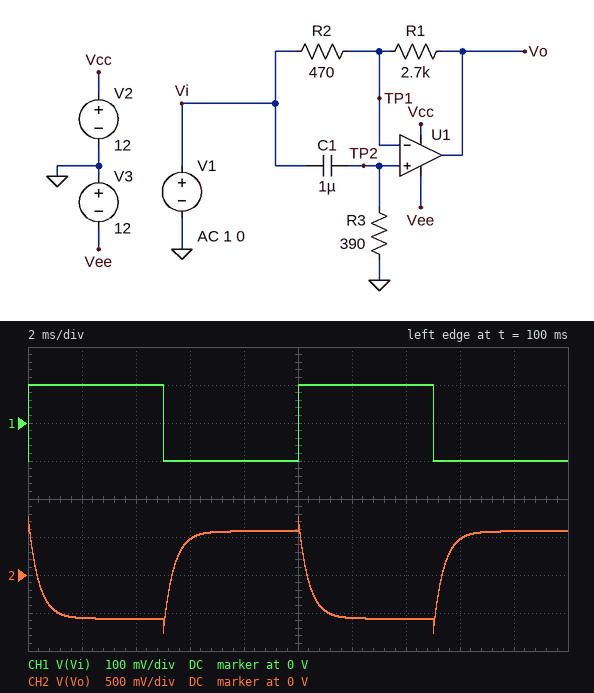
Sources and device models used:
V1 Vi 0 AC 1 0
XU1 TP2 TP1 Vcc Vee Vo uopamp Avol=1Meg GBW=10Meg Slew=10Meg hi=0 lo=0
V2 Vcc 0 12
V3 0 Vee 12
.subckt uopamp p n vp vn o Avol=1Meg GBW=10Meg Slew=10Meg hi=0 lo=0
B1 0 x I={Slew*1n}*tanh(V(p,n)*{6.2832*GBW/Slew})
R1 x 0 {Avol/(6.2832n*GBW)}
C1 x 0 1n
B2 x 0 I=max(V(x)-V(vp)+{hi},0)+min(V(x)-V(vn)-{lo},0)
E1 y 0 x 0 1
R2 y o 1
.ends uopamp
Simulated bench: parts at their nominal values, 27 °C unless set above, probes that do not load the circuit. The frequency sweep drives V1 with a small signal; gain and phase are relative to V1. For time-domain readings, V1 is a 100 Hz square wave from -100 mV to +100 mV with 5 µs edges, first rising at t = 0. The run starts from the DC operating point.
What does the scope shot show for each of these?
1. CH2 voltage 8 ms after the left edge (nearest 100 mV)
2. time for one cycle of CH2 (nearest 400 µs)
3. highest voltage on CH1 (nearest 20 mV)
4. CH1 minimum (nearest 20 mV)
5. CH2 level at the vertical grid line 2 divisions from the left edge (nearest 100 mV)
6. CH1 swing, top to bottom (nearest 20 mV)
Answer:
600 mV
10.0 ms
100 mV
-100 mV
-600 mV
200 mV
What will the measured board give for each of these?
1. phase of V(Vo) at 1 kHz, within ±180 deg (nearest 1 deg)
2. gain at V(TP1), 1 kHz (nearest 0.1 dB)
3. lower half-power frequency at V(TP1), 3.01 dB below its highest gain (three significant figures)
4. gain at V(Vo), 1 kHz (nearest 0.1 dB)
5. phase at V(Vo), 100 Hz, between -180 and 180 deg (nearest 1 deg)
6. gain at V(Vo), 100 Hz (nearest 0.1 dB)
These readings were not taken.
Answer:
89 deg
-0.7 dB
408 Hz
7.5 dB
164 deg
14.9 dB
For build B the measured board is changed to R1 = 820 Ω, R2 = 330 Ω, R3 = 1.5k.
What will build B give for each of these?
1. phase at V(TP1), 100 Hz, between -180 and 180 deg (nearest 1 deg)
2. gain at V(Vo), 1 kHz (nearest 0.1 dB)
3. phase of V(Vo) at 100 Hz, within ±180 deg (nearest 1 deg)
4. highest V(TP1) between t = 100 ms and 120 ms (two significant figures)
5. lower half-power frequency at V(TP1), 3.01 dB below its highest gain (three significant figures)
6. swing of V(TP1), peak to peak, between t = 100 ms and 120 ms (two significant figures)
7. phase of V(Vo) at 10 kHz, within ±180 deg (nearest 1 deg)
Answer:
47 deg
0.2 dB
116 deg
190 mV
106 Hz
390 mV
2 deg
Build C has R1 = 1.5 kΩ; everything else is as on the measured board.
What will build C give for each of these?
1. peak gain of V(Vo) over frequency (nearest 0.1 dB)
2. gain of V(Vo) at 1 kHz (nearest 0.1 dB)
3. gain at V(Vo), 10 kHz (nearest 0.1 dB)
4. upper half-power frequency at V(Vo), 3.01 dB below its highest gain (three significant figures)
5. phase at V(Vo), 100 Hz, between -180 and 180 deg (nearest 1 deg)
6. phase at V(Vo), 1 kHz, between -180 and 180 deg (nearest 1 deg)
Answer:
10.1 dB
3.6 dB
0.1 dB
455 Hz
162 deg
75 deg
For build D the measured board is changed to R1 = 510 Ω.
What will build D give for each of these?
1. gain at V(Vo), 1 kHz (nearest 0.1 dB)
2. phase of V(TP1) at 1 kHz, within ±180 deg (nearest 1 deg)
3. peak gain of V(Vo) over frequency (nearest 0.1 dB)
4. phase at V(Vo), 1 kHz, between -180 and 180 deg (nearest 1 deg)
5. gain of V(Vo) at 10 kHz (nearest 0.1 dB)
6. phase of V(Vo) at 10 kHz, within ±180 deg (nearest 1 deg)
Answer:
0.1 dB
22 deg
0.7 dB
46 deg
0 dB
5 deg
